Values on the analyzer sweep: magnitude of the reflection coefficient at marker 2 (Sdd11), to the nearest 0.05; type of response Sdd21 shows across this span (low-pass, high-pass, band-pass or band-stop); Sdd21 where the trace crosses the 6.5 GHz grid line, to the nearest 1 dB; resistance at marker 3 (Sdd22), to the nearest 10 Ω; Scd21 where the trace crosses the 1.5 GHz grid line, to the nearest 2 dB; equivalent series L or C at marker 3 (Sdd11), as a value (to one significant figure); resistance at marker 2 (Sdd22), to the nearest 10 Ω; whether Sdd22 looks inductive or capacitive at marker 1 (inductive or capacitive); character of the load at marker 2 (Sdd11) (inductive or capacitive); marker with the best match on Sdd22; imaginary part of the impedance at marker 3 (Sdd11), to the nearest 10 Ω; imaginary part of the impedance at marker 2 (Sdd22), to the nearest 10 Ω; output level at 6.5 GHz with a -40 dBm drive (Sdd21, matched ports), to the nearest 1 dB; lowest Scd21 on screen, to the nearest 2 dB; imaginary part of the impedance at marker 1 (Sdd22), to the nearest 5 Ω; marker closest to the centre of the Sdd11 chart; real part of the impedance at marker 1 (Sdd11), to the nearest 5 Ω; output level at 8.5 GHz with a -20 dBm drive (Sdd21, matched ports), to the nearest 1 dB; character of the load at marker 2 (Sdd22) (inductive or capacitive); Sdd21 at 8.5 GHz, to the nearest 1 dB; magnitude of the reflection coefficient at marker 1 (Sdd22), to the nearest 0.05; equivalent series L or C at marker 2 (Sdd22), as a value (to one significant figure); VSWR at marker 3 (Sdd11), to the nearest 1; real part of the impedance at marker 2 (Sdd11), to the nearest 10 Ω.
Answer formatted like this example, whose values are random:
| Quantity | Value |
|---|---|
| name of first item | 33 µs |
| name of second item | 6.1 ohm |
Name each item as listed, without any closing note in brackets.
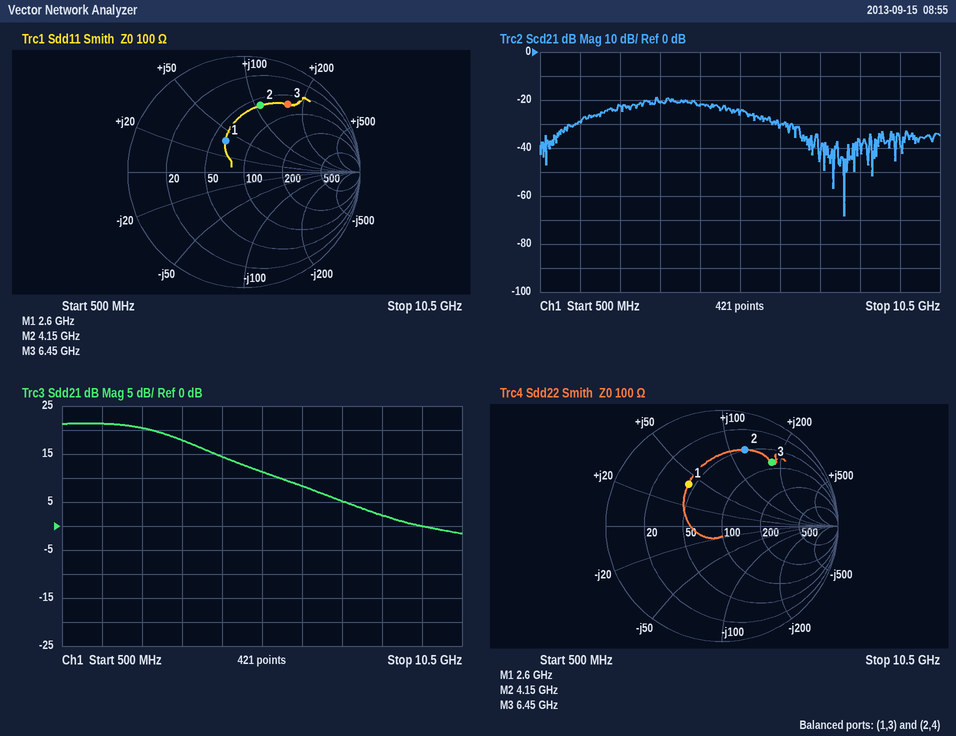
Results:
| Quantity | Value |
|---|---|
| magnitude of the reflection coefficient at marker 2 (Sdd11), to the nearest 0.05 | 0.60 |
| type of response Sdd21 shows across this span | low-pass |
| Sdd21 where the trace crosses the 6.5 GHz grid line, to the nearest 1 dB | 8 dB |
| resistance at marker 3 (Sdd22), to the nearest 10 Ω | 80 Ω |
| Scd21 where the trace crosses the 1.5 GHz grid line, to the nearest 2 dB | -30 dB |
| equivalent series L or C at marker 3 (Sdd11), as a value | 4 nH |
| resistance at marker 2 (Sdd22), to the nearest 10 Ω | 50 Ω |
| whether Sdd22 looks inductive or capacitive at marker 1 | inductive |
| character of the load at marker 2 (Sdd11) | inductive |
| marker with the best match on Sdd22 | marker 1 |
| imaginary part of the impedance at marker 3 (Sdd11), to the nearest 10 Ω | +160 Ω |
| imaginary part of the impedance at marker 2 (Sdd22), to the nearest 10 Ω | +120 Ω |
| output level at 6.5 GHz with a -40 dBm drive (Sdd21, matched ports), to the nearest 1 dB | -32 dBm |
| lowest Scd21 on screen, to the nearest 2 dB | -68 dB |
| imaginary part of the impedance at marker 1 (Sdd22), to the nearest 5 Ω | +40 Ω |
| marker closest to the centre of the Sdd11 chart | marker 1 |
| real part of the impedance at marker 1 (Sdd11), to the nearest 5 Ω | 65 Ω |
| output level at 8.5 GHz with a -20 dBm drive (Sdd21, matched ports), to the nearest 1 dB | -18 dBm |
| character of the load at marker 2 (Sdd22) | inductive |
| Sdd21 at 8.5 GHz, to the nearest 1 dB | 2 dB |
| magnitude of the reflection coefficient at marker 1 (Sdd22), to the nearest 0.05 | 0.45 |
| equivalent series L or C at marker 2 (Sdd22), as a value | 5 nH |
| VSWR at marker 3 (Sdd11), to the nearest 1 | 6 |
| real part of the impedance at marker 2 (Sdd11), to the nearest 10 Ω | 60 Ω |
